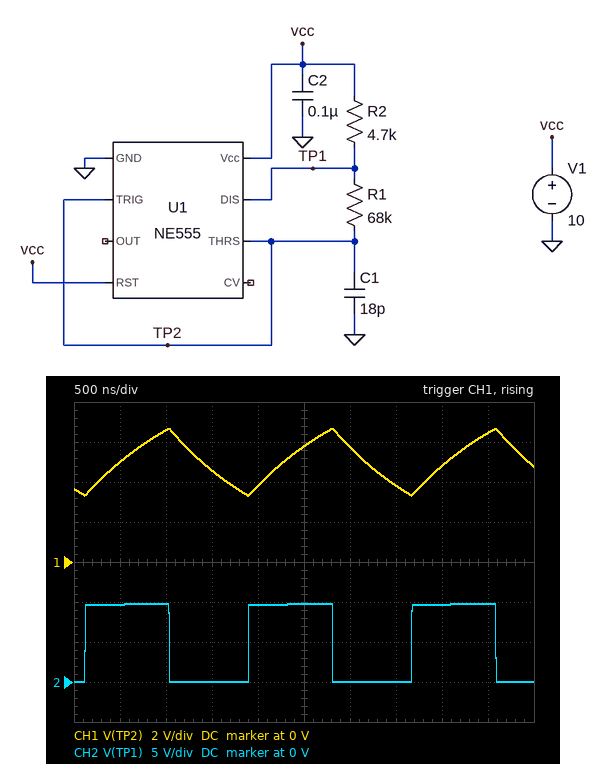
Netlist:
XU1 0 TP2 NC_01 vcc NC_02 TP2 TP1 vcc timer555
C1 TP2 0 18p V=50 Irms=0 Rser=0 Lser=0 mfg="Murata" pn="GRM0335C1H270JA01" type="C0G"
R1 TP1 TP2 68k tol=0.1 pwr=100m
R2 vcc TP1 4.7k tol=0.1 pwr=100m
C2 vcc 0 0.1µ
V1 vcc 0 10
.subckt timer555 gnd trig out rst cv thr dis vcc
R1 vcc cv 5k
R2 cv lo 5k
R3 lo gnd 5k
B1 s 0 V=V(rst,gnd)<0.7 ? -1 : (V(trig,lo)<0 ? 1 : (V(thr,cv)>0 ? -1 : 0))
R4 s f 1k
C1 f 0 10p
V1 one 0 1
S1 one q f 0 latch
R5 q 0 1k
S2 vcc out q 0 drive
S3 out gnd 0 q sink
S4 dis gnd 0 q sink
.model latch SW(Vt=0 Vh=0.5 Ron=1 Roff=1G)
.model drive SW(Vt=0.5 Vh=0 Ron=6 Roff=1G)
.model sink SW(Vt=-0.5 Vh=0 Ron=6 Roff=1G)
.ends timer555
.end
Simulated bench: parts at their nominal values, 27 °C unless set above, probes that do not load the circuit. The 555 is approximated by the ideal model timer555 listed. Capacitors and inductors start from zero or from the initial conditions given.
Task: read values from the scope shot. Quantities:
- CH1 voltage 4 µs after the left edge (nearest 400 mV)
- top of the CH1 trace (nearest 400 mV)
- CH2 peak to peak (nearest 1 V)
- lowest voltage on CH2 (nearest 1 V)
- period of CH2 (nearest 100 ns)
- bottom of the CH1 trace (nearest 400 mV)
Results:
4.8 V
6.8 V
10 V
0 V
1.8 µs
3.2 V
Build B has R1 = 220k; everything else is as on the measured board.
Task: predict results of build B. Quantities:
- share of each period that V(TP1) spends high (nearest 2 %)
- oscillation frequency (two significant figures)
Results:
50 %
180 kHz
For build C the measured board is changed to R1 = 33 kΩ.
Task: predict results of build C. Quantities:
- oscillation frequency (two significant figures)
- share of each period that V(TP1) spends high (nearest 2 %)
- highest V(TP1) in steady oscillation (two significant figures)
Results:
1.1 MHz
54 %
9.6 V
